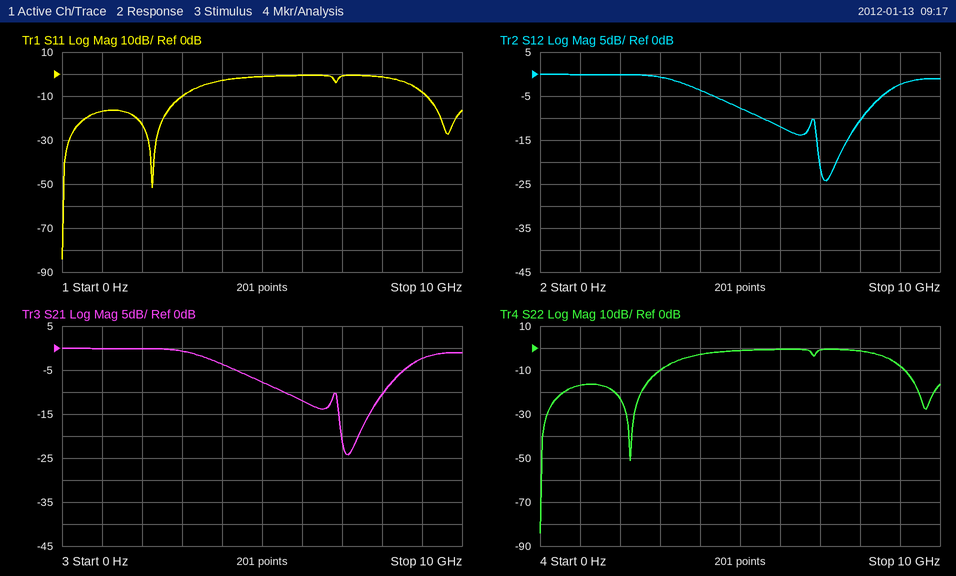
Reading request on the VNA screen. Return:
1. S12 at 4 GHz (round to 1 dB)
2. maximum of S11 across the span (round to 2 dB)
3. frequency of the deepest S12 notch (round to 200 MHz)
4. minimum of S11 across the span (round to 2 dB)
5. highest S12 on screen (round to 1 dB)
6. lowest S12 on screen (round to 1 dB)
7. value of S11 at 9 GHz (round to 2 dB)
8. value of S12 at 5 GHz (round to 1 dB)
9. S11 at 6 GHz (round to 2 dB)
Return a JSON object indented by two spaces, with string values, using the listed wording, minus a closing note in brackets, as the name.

{
  "S12 at 4 GHz": "-4 dB",
  "maximum of S11 across the span": "0 dB",
  "frequency of the deepest S12 notch": "7.2 GHz",
  "minimum of S11 across the span": "-84 dB",
  "highest S12 on screen": "0 dB",
  "lowest S12 on screen": "-24 dB",
  "value of S11 at 9 GHz": "-8 dB",
  "value of S12 at 5 GHz": "-8 dB",
  "S11 at 6 GHz": "0 dB"
}
